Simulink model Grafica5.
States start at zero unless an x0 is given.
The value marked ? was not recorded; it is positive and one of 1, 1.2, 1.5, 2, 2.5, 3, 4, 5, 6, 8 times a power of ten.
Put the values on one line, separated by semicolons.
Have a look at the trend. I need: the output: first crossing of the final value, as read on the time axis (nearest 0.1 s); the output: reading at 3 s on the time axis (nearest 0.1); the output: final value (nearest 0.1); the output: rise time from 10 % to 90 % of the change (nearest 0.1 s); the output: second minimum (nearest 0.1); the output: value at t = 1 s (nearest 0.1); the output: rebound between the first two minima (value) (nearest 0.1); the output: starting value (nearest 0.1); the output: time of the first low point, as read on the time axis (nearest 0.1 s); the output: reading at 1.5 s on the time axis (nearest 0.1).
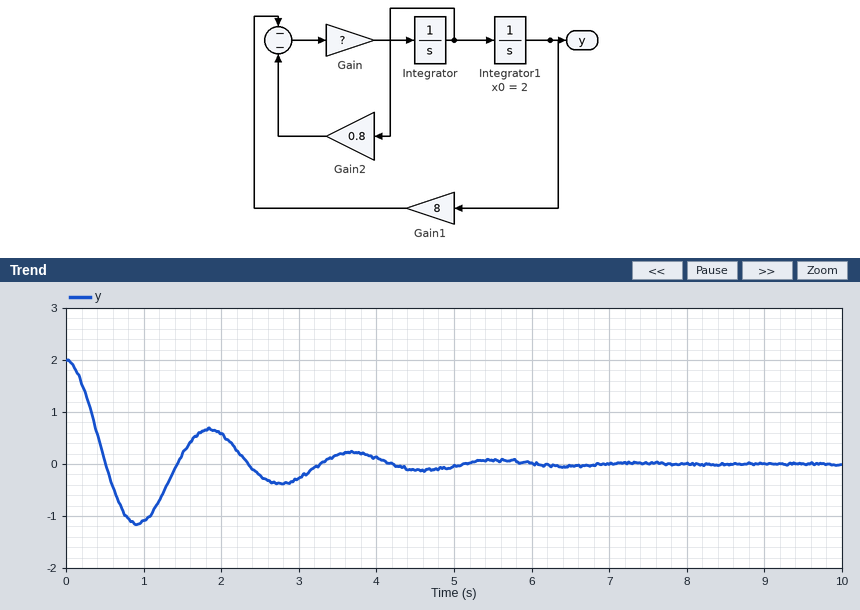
0.5 s; -0.3; 0.0; 0.3 s; -0.4; -1.1; 0.7; 2.0; 0.9 s; 0.2
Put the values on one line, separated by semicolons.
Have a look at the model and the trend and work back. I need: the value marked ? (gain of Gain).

1.5
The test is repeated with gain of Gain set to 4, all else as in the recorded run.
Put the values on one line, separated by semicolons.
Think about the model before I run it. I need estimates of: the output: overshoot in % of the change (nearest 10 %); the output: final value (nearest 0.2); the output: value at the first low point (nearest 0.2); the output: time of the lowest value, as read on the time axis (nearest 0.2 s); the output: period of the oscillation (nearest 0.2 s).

40 %; 0.0; -0.8; 0.6 s; 1.2 s
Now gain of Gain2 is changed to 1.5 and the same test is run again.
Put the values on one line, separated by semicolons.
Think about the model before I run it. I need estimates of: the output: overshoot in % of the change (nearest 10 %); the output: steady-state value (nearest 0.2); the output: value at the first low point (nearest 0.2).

30 %; 0.0; -0.6
